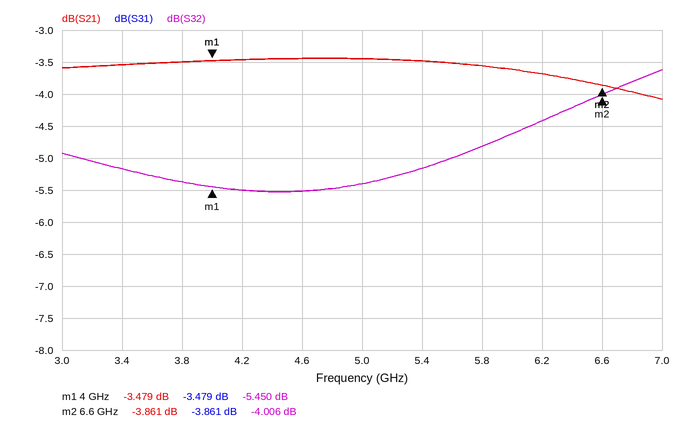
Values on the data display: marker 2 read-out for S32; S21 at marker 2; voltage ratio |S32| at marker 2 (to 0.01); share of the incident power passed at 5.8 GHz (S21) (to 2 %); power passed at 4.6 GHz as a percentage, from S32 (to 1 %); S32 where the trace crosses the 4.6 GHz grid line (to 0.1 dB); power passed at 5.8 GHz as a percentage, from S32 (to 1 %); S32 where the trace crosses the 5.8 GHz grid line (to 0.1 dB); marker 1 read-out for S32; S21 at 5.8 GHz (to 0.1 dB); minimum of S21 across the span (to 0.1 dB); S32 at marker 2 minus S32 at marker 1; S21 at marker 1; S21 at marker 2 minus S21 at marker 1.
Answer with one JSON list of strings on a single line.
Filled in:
["-4.006 dB", "-3.861 dB", "0.63", "44 %", "28 %", "-5.5 dB", "33 %", "-4.8 dB", "-5.450 dB", "-3.6 dB", "-4.1 dB", "1.444 dB", "-3.479 dB", "-0.382 dB"]
